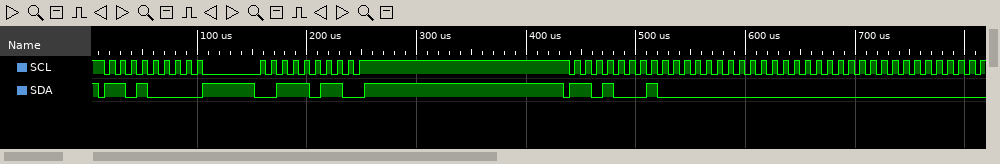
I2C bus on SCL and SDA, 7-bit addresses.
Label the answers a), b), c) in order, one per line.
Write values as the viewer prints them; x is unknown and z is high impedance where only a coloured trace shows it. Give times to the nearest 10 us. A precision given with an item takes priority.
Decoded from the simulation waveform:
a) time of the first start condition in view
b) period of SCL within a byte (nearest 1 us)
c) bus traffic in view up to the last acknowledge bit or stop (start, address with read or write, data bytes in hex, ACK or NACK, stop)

a) 10 us
b) 10 us
c) start, address 68 write ACK, 3B ACK, stop, start, address 68 read ACK, 00 ACK, 00 ACK, 00 ACK
